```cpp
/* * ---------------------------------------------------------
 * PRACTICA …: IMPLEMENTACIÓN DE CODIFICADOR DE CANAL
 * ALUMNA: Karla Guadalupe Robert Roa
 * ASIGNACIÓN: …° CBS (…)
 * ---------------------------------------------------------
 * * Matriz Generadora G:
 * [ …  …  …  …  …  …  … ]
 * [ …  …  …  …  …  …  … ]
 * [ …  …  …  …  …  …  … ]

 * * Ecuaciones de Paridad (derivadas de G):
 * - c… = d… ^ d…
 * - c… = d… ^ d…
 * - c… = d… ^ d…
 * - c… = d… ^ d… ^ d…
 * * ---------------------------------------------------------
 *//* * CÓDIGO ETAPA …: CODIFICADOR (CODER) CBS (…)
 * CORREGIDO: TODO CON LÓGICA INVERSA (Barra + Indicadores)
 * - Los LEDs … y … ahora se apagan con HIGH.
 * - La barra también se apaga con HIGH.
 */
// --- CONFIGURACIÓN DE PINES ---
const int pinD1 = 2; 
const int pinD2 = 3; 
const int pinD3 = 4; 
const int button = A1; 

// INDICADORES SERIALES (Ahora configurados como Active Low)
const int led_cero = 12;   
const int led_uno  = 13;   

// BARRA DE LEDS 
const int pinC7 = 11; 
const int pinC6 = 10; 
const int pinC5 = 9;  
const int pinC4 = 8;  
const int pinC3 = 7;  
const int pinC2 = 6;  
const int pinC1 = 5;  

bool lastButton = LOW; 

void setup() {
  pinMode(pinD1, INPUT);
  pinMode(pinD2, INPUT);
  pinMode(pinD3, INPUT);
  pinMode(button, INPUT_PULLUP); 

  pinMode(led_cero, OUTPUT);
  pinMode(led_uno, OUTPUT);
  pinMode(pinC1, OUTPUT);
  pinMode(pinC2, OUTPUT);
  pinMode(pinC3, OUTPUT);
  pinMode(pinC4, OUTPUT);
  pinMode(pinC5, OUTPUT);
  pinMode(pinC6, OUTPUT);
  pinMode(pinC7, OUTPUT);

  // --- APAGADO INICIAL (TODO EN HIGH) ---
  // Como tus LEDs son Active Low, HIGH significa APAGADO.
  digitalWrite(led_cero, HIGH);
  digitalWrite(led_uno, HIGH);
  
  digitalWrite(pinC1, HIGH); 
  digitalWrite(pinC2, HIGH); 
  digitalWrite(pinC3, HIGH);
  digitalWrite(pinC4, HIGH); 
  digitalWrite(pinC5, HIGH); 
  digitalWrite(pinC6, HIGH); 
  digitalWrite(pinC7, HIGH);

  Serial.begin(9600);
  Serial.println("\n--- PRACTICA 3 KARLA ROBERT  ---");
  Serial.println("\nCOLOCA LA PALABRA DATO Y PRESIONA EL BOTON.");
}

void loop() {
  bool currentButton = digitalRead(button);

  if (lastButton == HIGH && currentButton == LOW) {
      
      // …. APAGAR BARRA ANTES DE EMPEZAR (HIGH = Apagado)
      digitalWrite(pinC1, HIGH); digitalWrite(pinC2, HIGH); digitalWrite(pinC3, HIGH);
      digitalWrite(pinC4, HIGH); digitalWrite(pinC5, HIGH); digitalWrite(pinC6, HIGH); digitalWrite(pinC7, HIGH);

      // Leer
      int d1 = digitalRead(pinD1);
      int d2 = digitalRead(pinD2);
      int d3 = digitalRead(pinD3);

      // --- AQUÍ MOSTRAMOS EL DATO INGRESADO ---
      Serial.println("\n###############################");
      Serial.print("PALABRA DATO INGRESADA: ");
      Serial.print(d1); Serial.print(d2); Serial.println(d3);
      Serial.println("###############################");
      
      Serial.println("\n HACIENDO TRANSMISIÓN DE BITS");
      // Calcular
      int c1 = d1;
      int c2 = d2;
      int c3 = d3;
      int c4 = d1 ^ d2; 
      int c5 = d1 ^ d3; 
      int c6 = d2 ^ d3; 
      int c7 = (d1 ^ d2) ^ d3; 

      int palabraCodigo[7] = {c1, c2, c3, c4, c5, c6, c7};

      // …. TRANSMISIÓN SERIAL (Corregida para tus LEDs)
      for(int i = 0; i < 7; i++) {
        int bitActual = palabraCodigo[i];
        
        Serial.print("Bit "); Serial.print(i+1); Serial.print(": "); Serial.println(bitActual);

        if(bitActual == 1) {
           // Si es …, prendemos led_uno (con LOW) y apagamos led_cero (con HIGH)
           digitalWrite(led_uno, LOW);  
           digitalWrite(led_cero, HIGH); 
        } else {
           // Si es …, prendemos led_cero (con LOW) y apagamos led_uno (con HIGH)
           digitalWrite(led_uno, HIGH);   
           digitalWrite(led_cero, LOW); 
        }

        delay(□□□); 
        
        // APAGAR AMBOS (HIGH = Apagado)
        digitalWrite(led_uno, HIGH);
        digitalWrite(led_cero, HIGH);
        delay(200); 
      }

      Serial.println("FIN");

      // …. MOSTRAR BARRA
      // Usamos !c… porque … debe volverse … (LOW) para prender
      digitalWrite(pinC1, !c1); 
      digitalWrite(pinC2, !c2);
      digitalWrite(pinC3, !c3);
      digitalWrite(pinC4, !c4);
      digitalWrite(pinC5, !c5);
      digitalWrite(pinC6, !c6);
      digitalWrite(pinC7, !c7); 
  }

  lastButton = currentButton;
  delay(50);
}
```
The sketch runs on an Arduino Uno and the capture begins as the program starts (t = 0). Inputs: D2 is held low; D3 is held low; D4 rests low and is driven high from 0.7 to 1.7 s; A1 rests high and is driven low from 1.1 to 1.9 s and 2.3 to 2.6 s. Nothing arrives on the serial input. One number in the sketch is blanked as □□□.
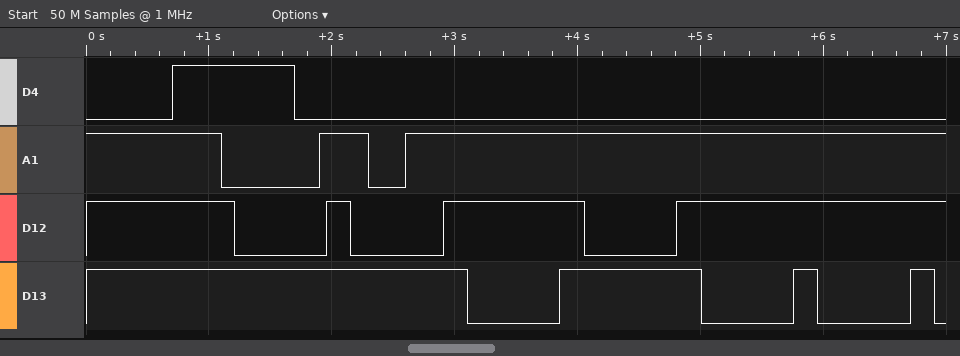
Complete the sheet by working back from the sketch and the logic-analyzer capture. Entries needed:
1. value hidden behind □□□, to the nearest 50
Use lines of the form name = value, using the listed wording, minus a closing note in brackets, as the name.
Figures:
value hidden behind □□□, to the nearest 50 = 750
